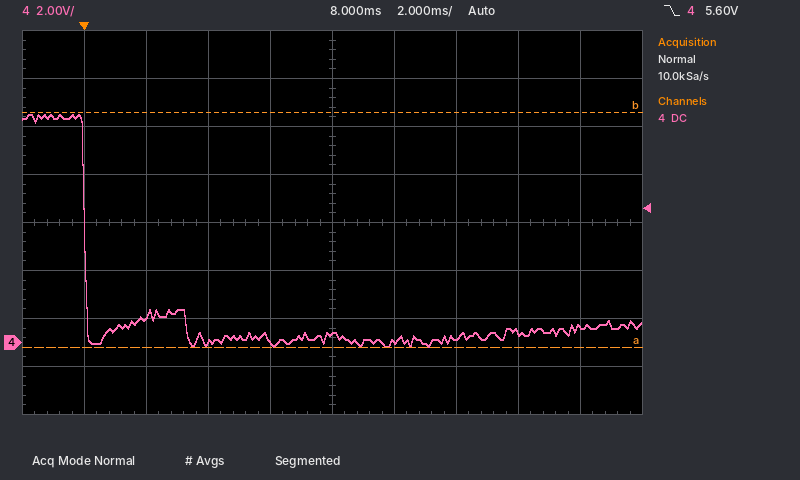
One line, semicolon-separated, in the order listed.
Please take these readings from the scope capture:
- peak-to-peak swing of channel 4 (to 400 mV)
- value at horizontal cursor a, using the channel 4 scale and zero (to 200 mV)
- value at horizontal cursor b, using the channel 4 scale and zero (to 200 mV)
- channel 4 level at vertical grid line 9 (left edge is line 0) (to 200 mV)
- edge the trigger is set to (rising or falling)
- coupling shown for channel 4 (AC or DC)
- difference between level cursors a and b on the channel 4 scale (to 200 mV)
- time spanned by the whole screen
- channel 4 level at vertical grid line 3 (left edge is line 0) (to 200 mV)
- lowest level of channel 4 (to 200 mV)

9.6 V; -200 mV; 9.6 V; 600 mV; falling; DC; 9.8 V; 20 ms; 0.0 V; -200 mV
